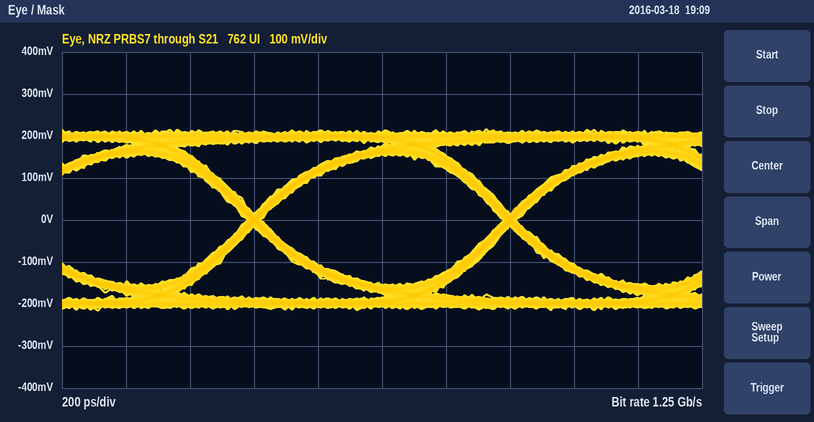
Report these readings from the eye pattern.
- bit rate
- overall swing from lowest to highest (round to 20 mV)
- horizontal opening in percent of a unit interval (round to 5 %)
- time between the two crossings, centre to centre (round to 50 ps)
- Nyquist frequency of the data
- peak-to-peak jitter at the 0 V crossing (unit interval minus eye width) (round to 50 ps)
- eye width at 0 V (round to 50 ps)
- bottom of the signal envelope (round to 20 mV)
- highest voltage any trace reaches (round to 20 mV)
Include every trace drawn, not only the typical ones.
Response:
1.25 Gb/s
440 mV
95 %
800 ps
625 MHz
50 ps
750 ps
-220 mV
220 mV
